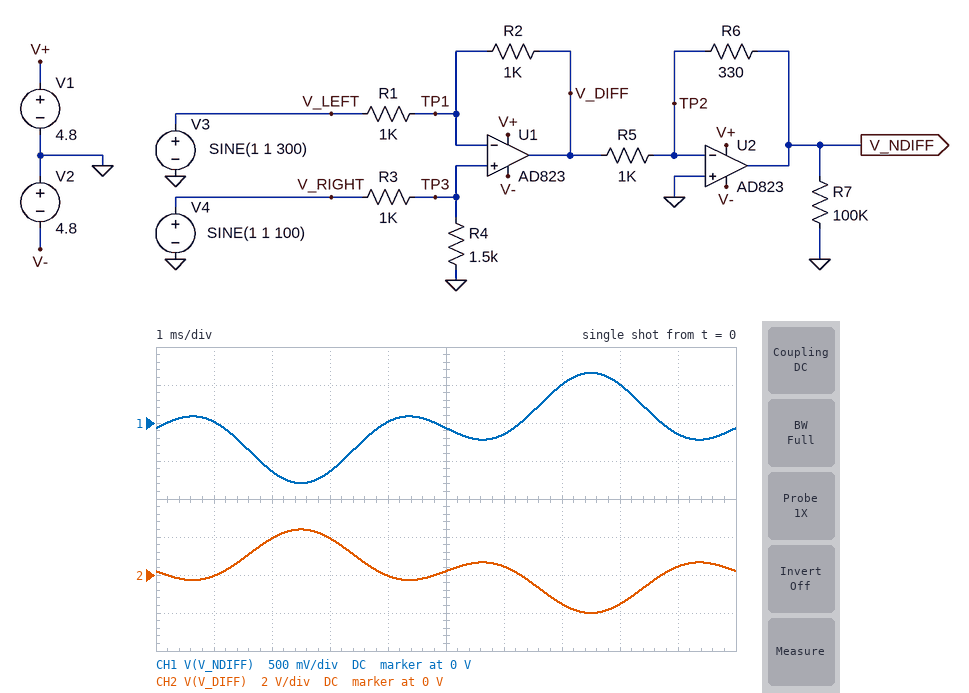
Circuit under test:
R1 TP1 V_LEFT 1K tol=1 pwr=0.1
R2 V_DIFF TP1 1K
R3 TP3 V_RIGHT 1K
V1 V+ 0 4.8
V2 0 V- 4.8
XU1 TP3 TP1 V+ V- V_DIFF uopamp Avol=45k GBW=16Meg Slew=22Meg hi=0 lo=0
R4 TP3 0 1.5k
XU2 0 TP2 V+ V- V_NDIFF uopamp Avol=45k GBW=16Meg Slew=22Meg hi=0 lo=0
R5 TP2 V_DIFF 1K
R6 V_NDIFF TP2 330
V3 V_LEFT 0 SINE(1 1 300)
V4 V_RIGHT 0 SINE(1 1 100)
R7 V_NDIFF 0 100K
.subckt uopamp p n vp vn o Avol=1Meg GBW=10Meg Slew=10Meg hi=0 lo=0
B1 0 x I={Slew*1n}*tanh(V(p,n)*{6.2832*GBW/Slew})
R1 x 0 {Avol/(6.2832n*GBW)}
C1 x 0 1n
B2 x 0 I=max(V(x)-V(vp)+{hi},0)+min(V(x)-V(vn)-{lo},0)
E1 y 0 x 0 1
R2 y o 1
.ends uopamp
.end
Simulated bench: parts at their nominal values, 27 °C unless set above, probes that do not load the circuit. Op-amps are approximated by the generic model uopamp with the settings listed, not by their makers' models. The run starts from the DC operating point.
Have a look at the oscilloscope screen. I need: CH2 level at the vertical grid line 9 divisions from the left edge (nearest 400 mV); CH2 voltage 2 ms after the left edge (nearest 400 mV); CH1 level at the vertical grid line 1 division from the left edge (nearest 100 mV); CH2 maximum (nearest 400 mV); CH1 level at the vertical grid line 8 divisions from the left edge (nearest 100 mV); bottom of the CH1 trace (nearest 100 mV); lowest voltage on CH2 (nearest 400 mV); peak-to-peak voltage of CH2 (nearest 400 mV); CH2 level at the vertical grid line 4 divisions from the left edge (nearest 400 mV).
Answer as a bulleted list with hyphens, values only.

- 400 mV
- 2.0 V
- 0 V
- 2.4 V
- 500 mV
- -800 mV
- -2.0 V
- 4.4 V
- 0 V
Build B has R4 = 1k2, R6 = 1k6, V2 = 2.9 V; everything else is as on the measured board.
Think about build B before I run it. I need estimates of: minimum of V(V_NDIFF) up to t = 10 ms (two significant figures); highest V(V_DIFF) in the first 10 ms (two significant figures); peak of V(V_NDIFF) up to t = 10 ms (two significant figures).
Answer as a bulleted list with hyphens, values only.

- -2.9 V
- 2.2 V
- 3.2 V
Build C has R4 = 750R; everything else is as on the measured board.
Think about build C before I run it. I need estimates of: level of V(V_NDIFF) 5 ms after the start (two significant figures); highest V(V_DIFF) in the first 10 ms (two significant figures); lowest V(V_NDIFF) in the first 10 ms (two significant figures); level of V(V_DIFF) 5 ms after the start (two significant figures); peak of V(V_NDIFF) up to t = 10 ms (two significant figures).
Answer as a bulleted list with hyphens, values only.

- 47 mV
- 1.7 V
- -570 mV
- -140 mV
- 660 mV
